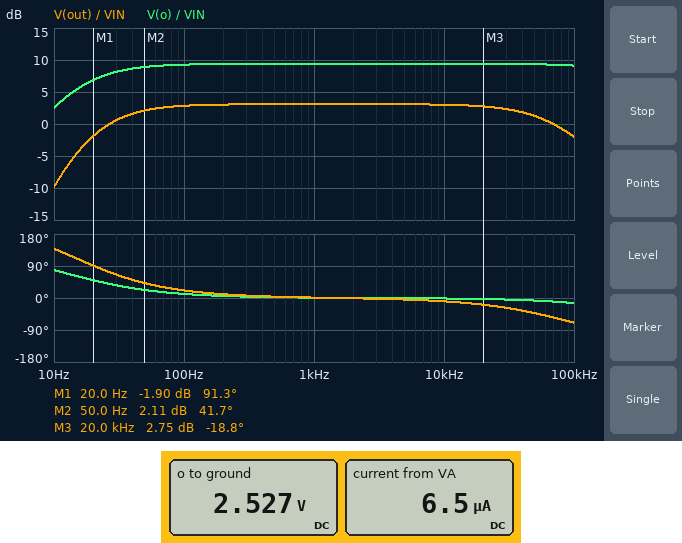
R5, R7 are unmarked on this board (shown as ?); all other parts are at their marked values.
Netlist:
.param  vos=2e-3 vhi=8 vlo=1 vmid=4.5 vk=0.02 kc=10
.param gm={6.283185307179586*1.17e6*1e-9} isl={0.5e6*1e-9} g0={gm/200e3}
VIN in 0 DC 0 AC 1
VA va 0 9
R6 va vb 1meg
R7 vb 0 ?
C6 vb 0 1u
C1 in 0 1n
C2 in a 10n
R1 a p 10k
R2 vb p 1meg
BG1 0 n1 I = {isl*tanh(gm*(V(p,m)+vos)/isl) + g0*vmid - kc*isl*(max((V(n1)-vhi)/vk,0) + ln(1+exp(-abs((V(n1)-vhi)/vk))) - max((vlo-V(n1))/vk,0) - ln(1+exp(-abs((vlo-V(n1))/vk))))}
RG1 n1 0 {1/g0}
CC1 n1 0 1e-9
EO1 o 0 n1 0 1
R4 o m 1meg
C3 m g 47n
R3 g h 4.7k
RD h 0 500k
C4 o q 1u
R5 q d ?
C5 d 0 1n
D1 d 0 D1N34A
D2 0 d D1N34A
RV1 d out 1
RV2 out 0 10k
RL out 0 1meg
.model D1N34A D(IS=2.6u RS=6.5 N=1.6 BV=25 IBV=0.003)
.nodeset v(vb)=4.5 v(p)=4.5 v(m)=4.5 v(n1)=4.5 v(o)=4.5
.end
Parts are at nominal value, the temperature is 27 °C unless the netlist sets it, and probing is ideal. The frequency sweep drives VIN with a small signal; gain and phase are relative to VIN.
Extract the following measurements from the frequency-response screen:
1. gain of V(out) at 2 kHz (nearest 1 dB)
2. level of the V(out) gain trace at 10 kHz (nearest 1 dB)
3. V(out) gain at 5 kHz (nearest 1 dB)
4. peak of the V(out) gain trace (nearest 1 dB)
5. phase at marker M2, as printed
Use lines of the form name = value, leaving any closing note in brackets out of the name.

gain of V(out) at 2 kHz = 3 dB
level of the V(out) gain trace at 10 kHz = 3 dB
V(out) gain at 5 kHz = 3 dB
peak of the V(out) gain trace = 3 dB
phase at marker M2, as printed = 41.7 deg
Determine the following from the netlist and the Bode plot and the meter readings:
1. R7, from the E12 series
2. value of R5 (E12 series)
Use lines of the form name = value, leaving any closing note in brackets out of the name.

R7, from the E12 series = 390 kΩ
value of R5 = 4.7 kΩ
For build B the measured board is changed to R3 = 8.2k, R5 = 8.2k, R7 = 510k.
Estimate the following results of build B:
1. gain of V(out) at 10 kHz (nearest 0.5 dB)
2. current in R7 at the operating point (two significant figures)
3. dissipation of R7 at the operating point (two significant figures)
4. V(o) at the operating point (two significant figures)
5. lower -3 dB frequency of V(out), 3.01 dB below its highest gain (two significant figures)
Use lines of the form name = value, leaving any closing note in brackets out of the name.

gain of V(out) at 10 kHz = 0 dB
current in R7 at the operating point = 6.0 µA
dissipation of R7 at the operating point = 18 µW
V(o) at the operating point = 3.0 V
lower -3 dB frequency of V(out), 3.01 dB below its highest gain = 24 Hz
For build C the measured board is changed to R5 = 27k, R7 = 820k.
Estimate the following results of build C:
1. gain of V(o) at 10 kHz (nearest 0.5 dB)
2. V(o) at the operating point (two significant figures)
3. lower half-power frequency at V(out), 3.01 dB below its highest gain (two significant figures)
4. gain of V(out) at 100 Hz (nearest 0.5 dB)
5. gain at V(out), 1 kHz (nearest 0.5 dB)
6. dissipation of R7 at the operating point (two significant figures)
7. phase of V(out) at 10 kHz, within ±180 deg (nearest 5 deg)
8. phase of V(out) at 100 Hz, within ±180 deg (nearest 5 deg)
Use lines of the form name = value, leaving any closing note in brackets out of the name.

gain of V(o) at 10 kHz = 9.5 dB
V(o) at the operating point = 4.1 V
lower half-power frequency at V(out), 3.01 dB below its highest gain = 19 Hz
gain of V(out) at 100 Hz = -8.0 dB
gain at V(out), 1 kHz = -7.5 dB
dissipation of R7 at the operating point = 20 µW
phase of V(out) at 10 kHz, within ±180 deg = -15 deg
phase of V(out) at 100 Hz, within ±180 deg = 15 deg
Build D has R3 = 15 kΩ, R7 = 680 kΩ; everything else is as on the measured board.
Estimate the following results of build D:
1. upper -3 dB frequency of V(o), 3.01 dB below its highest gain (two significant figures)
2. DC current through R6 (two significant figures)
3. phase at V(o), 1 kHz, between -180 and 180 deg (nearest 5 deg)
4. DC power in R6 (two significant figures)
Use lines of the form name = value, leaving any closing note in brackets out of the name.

upper -3 dB frequency of V(o), 3.01 dB below its highest gain = 400 kHz
DC current through R6 = 5.4 µA
phase at V(o), 1 kHz, between -180 and 180 deg = 0 deg
DC power in R6 = 29 µW
